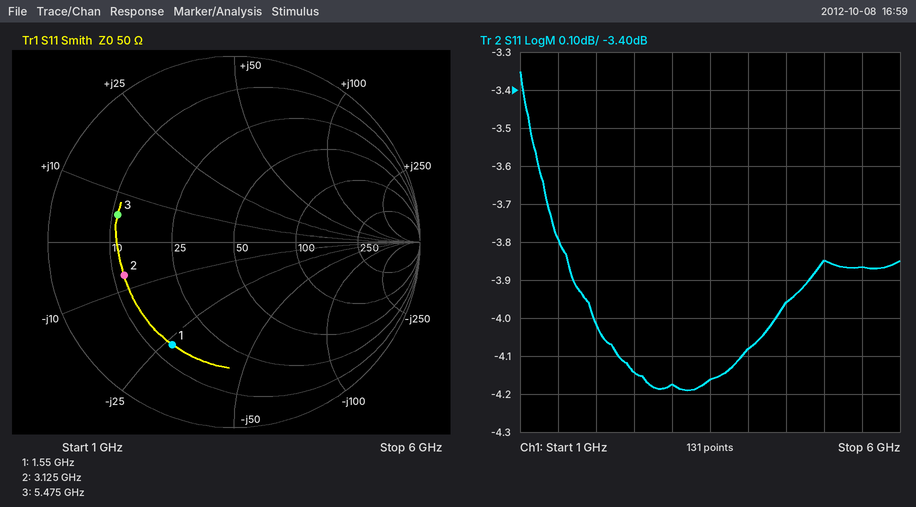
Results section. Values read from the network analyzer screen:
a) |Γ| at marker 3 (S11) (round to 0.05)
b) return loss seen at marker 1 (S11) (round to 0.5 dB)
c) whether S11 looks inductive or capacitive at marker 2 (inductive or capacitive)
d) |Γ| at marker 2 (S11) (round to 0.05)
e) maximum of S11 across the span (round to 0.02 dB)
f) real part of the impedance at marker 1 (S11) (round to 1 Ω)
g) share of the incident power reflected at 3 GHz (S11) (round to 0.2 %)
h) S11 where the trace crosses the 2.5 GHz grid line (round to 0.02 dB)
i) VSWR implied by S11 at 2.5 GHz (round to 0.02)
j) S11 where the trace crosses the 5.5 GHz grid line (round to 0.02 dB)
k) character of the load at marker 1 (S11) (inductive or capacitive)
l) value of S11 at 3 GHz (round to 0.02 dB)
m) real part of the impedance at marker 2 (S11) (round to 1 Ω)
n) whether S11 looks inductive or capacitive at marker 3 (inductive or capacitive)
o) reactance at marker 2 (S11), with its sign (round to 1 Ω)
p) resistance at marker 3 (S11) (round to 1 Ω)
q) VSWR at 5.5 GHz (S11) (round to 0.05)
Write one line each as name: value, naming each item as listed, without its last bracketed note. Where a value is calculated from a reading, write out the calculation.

|Γ| at marker 3 (S11): 0.65
return loss seen at marker 1 (S11): 4.0 dB
whether S11 looks inductive or capacitive at marker 2: capacitive
|Γ| at marker 2 (S11): 0.60
maximum of S11 across the span: -3.36 dB
real part of the impedance at marker 1 (S11): 14 Ω
share of the incident power reflected at 3 GHz (S11): 10^(-4.18/10) ≈ 38.2 %
S11 where the trace crosses the 2.5 GHz grid line: -4.14 dB
VSWR implied by S11 at 2.5 GHz: |Γ| = 10^(-4.14/20) = 0.6209; VSWR = (1 + 0.6209)/(1 − 0.6209) ≈ 4.28
S11 where the trace crosses the 5.5 GHz grid line: -3.86 dB
character of the load at marker 1 (S11): capacitive
value of S11 at 3 GHz: -4.18 dB
real part of the impedance at marker 2 (S11): 12 Ω
whether S11 looks inductive or capacitive at marker 3: inductive
reactance at marker 2 (S11), with its sign: -7 Ω
resistance at marker 3 (S11): 11 Ω
VSWR at 5.5 GHz (S11): |Γ| = 10^(-3.86/20) = 0.6412; VSWR = (1 + 0.6412)/(1 − 0.6412) ≈ 4.57, so 4.55 to the nearest 0.05
